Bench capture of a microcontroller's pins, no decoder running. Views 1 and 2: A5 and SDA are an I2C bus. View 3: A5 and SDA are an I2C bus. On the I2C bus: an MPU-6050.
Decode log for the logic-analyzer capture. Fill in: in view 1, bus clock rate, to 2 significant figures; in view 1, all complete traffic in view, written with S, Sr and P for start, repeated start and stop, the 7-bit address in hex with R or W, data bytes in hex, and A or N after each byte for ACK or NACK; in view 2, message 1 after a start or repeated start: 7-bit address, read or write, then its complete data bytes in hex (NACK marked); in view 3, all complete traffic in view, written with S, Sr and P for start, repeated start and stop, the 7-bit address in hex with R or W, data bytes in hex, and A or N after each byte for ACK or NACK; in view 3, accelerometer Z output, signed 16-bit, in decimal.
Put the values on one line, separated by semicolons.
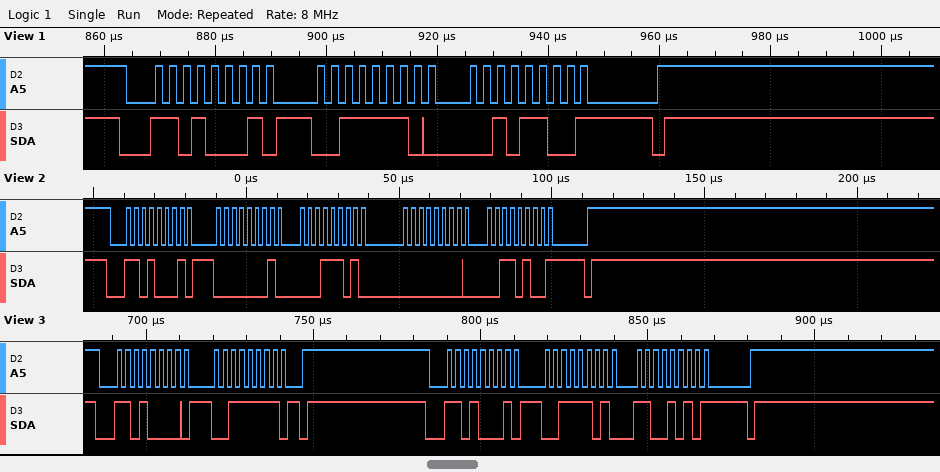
400 kHz; S 68R A 3E A 2C N P; 0x68 read: 01 1D 00 34 NACK; S 68W A 3F A P S 68R A 3D A CA N P; 15818
